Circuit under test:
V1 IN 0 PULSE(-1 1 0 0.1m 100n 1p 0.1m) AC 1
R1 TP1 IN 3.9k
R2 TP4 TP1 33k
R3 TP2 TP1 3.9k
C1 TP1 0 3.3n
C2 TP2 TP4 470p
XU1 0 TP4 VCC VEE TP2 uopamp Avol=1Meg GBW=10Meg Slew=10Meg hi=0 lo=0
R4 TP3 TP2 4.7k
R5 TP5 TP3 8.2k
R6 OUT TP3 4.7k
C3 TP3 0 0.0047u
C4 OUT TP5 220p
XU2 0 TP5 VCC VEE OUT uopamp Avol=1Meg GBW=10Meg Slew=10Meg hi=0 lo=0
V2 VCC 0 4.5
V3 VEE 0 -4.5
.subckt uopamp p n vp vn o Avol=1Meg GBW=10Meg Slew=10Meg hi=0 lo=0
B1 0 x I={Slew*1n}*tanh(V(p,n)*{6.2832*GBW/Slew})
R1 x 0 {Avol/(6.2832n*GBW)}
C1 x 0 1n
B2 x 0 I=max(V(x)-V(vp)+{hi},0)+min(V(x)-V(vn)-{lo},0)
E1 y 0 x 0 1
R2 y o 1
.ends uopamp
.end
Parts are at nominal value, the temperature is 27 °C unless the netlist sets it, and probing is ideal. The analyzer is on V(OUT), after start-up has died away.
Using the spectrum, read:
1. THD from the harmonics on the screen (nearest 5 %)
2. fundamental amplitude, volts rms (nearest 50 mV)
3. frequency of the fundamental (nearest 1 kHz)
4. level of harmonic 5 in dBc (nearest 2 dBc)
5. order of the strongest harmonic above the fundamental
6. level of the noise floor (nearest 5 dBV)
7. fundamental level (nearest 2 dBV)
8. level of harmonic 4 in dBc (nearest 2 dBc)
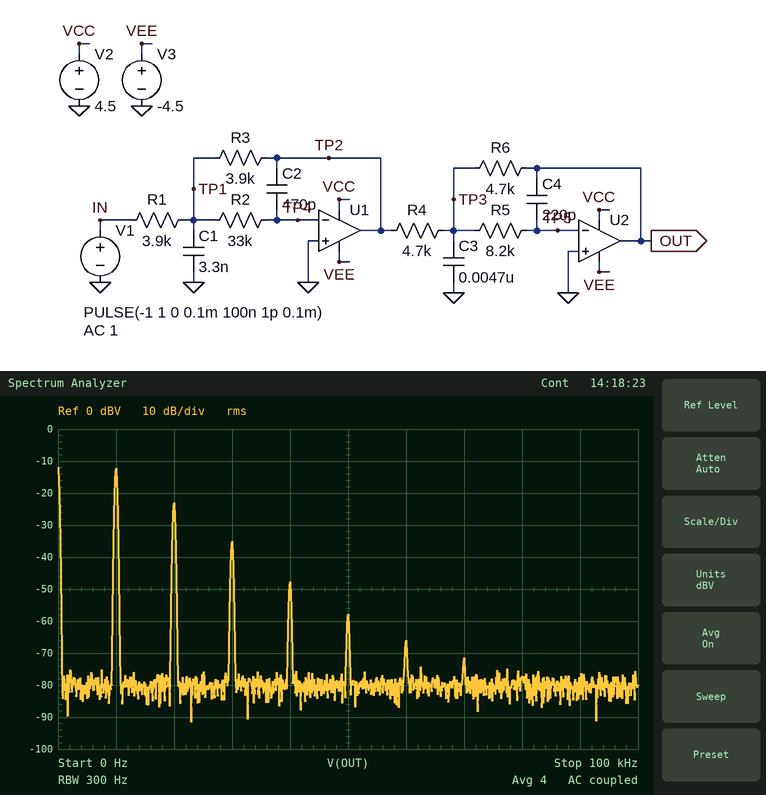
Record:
30 %
250 mV
10 kHz
-46 dBc
2
-80 dBV
-12 dBV
-36 dBc
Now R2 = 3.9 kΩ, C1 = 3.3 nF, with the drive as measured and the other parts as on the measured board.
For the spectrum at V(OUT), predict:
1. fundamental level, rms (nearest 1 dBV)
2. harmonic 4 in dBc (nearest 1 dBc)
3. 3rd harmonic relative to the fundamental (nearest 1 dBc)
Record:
-6 dBV
-22 dBc
-11 dBc
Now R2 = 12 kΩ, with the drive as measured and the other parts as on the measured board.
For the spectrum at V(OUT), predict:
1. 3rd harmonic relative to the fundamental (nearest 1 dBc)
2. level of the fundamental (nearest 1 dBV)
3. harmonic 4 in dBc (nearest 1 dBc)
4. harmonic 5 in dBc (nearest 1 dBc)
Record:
-19 dBc
-7 dBV
-32 dBc
-42 dBc
